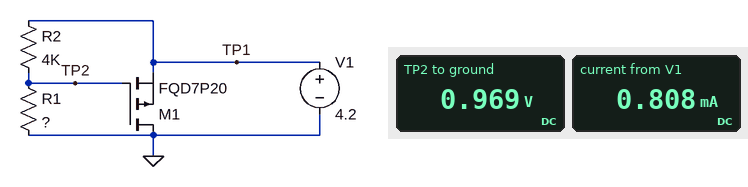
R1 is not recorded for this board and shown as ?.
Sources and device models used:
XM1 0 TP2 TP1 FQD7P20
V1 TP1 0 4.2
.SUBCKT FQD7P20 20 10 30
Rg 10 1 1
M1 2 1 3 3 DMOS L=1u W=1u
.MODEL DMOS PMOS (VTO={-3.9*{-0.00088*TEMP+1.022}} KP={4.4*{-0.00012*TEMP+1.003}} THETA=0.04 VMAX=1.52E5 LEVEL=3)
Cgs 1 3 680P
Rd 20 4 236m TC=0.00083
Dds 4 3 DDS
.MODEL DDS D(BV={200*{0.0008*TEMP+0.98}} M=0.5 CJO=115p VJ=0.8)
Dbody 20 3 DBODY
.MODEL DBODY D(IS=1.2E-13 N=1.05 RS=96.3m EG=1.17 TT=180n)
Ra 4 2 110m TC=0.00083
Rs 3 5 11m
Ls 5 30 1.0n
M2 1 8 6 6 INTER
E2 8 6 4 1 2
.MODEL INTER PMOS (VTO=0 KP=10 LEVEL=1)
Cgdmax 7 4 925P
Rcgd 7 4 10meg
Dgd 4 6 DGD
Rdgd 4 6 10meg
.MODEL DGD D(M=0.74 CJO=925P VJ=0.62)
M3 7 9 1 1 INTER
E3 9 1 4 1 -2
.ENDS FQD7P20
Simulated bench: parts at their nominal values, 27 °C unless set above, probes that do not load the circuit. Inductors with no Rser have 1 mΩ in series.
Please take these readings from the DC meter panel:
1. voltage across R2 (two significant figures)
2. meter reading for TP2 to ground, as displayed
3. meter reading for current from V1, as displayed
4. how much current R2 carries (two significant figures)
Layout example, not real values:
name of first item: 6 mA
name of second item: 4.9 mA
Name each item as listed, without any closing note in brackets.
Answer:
voltage across R2: 3.2 V
meter reading for TP2 to ground, as displayed: 0.969 V
meter reading for current from V1, as displayed: 0.808 mA
how much current R2 carries: 810 µA
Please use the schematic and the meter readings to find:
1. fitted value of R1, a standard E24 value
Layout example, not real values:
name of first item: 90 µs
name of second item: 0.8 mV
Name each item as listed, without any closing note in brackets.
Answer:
fitted value of R1, a standard E24 value: 1.2 kΩ
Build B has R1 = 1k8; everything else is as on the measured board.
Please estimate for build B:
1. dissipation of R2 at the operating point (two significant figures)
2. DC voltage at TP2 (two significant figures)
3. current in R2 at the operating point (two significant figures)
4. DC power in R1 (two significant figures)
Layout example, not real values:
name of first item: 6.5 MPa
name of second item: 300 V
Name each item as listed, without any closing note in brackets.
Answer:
dissipation of R2 at the operating point: 2.1 mW
DC voltage at TP2: 1.3 V
current in R2 at the operating point: 720 µA
DC power in R1: 940 µW
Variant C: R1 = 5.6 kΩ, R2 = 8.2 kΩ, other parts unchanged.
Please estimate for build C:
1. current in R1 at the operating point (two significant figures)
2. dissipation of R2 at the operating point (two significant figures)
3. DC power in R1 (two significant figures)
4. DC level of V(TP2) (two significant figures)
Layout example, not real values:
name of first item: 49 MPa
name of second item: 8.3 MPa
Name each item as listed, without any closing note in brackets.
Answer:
current in R1 at the operating point: 300 µA
dissipation of R2 at the operating point: 760 µW
DC power in R1: 520 µW
DC level of V(TP2): 1.7 V
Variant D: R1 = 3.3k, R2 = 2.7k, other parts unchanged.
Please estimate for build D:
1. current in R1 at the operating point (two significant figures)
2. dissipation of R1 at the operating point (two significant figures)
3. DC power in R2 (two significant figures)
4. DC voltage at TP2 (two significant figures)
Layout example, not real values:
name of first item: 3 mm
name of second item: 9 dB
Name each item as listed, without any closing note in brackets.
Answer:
current in R1 at the operating point: 700 µA
dissipation of R1 at the operating point: 1.6 mW
DC power in R2: 1.3 mW
DC voltage at TP2: 2.3 V
